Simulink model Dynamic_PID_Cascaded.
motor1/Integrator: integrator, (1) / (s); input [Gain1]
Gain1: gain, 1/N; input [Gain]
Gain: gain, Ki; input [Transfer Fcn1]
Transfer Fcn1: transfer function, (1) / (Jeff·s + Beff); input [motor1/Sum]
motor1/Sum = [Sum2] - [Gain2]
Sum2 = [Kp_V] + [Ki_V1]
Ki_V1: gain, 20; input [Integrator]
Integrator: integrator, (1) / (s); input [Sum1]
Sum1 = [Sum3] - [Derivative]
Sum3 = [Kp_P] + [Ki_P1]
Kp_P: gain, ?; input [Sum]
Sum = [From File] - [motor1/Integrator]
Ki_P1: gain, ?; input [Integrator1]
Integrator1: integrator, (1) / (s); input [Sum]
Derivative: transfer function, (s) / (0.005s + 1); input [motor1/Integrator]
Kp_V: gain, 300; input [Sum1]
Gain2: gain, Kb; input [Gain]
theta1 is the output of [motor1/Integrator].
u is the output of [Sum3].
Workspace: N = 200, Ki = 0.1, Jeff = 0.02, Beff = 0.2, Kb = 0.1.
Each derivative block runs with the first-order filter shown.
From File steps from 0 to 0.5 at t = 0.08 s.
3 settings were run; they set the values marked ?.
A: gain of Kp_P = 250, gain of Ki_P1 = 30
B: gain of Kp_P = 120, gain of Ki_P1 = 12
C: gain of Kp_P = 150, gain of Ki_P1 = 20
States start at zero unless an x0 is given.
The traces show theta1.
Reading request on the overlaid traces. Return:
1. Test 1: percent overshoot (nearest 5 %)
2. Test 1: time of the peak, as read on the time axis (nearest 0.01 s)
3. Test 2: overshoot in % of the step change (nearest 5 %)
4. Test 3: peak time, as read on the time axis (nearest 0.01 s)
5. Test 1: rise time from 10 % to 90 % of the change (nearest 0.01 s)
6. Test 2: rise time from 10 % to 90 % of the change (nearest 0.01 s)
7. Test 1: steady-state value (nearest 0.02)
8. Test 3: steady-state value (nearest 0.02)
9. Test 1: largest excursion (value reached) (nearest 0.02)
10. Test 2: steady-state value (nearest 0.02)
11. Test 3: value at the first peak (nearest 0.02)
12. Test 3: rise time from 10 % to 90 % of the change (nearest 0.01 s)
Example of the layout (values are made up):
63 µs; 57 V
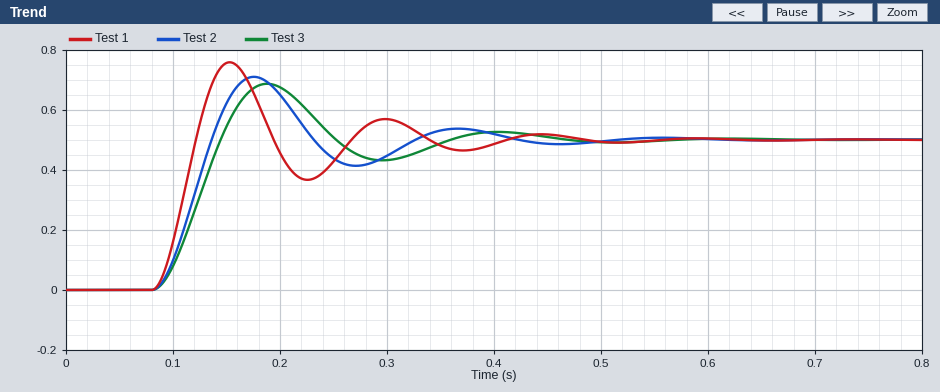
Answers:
50 %; 0.15 s; 40 %; 0.19 s; 0.03 s; 0.04 s; 0.50; 0.50; 0.76; 0.50; 0.68; 0.04 s
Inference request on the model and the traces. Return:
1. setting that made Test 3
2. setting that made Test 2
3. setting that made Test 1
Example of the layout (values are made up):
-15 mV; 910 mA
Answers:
B; C; A
